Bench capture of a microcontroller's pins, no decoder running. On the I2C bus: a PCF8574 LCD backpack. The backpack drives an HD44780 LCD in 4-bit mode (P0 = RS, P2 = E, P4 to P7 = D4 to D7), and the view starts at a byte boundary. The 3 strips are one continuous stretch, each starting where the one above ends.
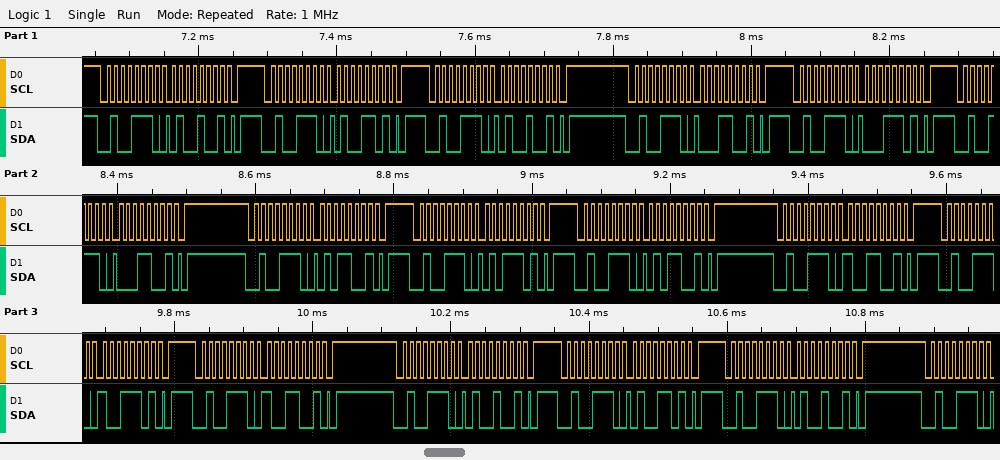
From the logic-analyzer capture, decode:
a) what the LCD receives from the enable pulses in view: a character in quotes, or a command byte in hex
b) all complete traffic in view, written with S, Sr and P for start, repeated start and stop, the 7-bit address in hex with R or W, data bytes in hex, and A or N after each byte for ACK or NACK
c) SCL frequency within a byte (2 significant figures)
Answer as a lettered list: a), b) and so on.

a) 'A' 'Y'
b) S 27W A 49 A P S 27W A 4D A P S 27W A 49 A P S 27W A 19 A P S 27W A 1D A P S 27W A 19 A P S 27W A 59 A P S 27W A 5D A P S 27W A 59 A P S 27W A 99 A P S 27W A 9D A P S 27W A 99 A P S 27W A 49 A P S 27W A 4D A P S 27W A 49 A P S 27W A
c) 100 kHz
